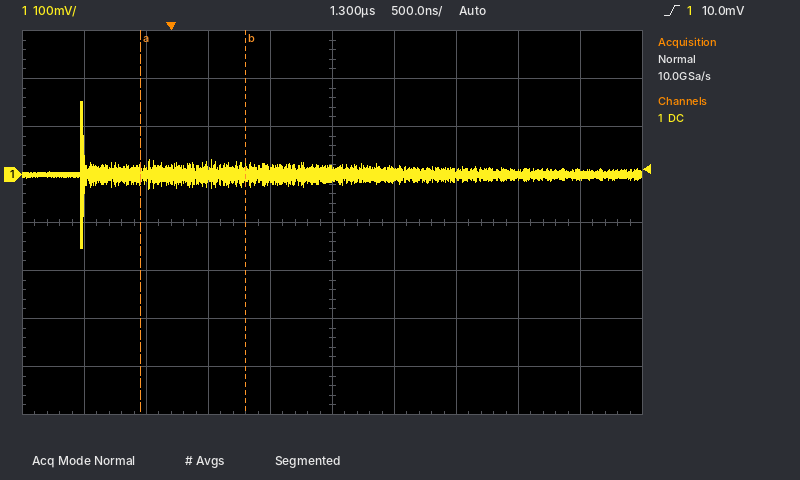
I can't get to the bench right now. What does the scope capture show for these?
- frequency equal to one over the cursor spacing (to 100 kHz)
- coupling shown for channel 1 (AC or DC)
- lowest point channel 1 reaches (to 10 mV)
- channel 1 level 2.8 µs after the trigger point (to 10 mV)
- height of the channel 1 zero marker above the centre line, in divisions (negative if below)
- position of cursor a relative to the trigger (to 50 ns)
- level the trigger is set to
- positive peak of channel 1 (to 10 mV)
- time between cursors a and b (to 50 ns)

1.2 MHz
DC
-150 mV
0 mV
+1.0 div
-250 ns
10.0 mV
150 mV
850 ns
